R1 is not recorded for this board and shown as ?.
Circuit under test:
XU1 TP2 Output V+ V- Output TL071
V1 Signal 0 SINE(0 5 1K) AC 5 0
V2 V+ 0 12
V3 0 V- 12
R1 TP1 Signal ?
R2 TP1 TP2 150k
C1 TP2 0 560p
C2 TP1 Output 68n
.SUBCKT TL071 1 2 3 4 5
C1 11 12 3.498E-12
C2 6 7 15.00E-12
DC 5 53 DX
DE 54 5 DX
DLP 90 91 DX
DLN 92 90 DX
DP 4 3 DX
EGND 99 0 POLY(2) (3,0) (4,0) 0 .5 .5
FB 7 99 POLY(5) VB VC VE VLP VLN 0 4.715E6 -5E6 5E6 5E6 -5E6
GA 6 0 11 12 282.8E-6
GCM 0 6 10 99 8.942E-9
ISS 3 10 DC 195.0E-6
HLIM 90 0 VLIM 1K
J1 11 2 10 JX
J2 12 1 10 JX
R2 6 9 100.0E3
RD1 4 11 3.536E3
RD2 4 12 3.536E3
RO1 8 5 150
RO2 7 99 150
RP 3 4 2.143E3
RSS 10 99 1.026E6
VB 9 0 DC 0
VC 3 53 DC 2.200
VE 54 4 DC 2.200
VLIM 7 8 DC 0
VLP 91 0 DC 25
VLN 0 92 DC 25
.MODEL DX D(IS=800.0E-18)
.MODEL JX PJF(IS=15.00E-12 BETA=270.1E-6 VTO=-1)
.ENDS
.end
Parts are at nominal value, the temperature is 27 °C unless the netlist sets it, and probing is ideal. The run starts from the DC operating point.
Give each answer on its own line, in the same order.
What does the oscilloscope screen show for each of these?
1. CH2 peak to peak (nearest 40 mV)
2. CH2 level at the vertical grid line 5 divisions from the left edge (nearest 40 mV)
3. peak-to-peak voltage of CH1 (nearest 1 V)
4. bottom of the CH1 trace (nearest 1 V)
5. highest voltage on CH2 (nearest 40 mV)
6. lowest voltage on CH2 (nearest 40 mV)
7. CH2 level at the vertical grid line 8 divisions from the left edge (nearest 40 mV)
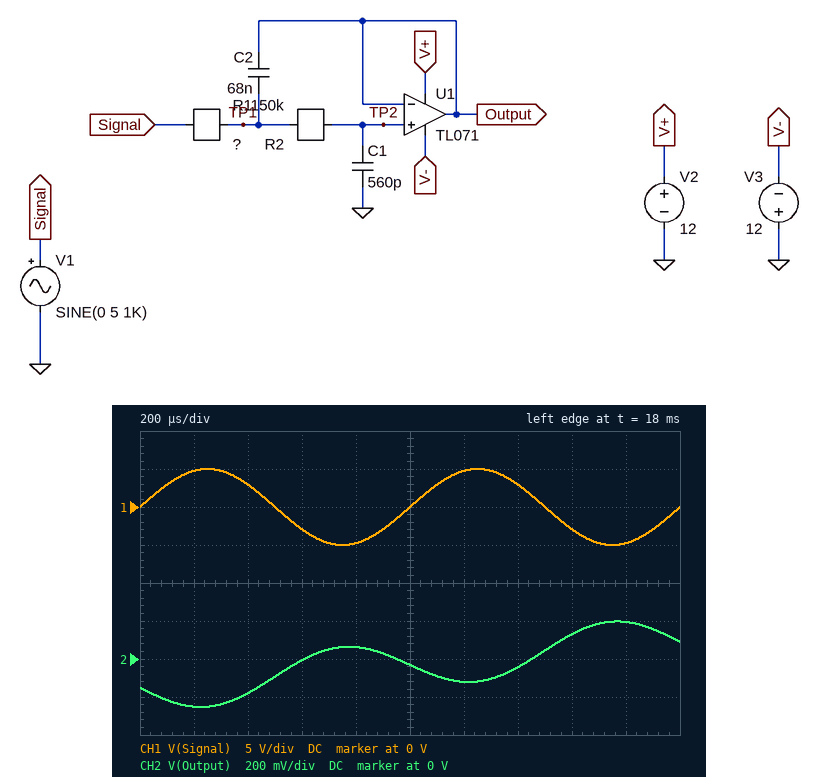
440 mV
-40 mV
10 V
-5 V
200 mV
-240 mV
120 mV
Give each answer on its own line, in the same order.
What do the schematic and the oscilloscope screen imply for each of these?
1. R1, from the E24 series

180 kΩ
